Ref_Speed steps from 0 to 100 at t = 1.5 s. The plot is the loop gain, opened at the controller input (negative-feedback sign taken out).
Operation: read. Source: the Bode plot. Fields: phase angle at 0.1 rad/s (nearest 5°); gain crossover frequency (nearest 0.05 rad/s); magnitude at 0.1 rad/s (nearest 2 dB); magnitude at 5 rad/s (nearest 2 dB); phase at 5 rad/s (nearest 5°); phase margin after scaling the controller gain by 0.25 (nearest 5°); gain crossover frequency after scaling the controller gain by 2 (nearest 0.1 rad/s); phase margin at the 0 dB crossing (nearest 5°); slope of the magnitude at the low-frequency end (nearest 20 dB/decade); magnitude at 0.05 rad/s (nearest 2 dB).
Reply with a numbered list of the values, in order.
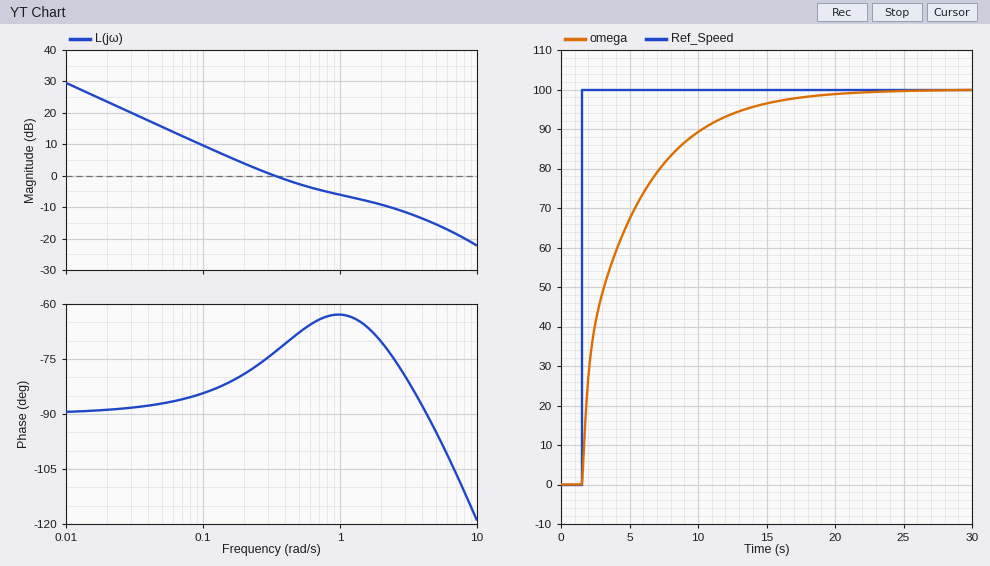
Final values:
1. -85°
2. 0.35 rad/s
3. 10 dB
4. -16 dB
5. -95°
6. 95°
7. 1.0 rad/s
8. 105°
9. -20 dB/decade
10. 16 dB
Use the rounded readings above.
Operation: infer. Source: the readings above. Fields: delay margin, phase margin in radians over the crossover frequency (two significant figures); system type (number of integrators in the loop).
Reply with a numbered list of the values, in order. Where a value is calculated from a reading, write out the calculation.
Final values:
1. 105 × π / 180 / 0.35 = 5.2 s
2. 1
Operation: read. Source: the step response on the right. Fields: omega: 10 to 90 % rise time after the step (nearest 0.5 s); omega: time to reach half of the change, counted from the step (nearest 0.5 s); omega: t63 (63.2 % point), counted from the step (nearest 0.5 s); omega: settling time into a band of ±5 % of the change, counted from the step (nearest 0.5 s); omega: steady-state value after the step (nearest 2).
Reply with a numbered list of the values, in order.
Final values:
1. 8.5 s
2. 1.5 s
3. 3.0 s
4. 12.0 s
5. 100
